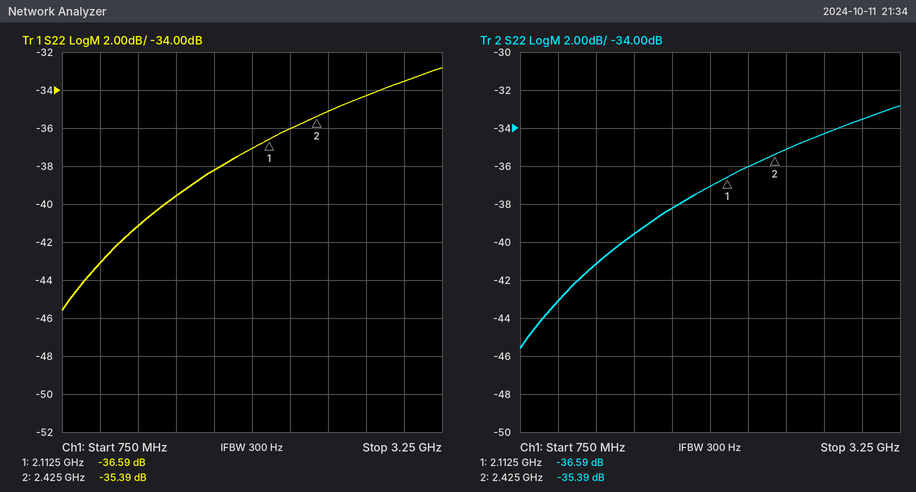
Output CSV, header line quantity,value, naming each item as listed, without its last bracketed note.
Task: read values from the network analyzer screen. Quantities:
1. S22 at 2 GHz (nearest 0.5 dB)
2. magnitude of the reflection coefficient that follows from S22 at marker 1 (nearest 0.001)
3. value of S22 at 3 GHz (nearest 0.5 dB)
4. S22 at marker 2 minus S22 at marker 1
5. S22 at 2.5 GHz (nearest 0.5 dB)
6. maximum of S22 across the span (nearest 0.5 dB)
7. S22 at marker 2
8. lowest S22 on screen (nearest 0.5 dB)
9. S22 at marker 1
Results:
quantity,value
S22 at 2 GHz,-37.0 dB
magnitude of the reflection coefficient that follows from S22 at marker 1,0.015
value of S22 at 3 GHz,-33.5 dB
S22 at marker 2 minus S22 at marker 1,1.20 dB
S22 at 2.5 GHz,-35.0 dB
maximum of S22 across the span,-33.0 dB
S22 at marker 2,-35.39 dB
lowest S22 on screen,-45.5 dB
S22 at marker 1,-36.59 dB
